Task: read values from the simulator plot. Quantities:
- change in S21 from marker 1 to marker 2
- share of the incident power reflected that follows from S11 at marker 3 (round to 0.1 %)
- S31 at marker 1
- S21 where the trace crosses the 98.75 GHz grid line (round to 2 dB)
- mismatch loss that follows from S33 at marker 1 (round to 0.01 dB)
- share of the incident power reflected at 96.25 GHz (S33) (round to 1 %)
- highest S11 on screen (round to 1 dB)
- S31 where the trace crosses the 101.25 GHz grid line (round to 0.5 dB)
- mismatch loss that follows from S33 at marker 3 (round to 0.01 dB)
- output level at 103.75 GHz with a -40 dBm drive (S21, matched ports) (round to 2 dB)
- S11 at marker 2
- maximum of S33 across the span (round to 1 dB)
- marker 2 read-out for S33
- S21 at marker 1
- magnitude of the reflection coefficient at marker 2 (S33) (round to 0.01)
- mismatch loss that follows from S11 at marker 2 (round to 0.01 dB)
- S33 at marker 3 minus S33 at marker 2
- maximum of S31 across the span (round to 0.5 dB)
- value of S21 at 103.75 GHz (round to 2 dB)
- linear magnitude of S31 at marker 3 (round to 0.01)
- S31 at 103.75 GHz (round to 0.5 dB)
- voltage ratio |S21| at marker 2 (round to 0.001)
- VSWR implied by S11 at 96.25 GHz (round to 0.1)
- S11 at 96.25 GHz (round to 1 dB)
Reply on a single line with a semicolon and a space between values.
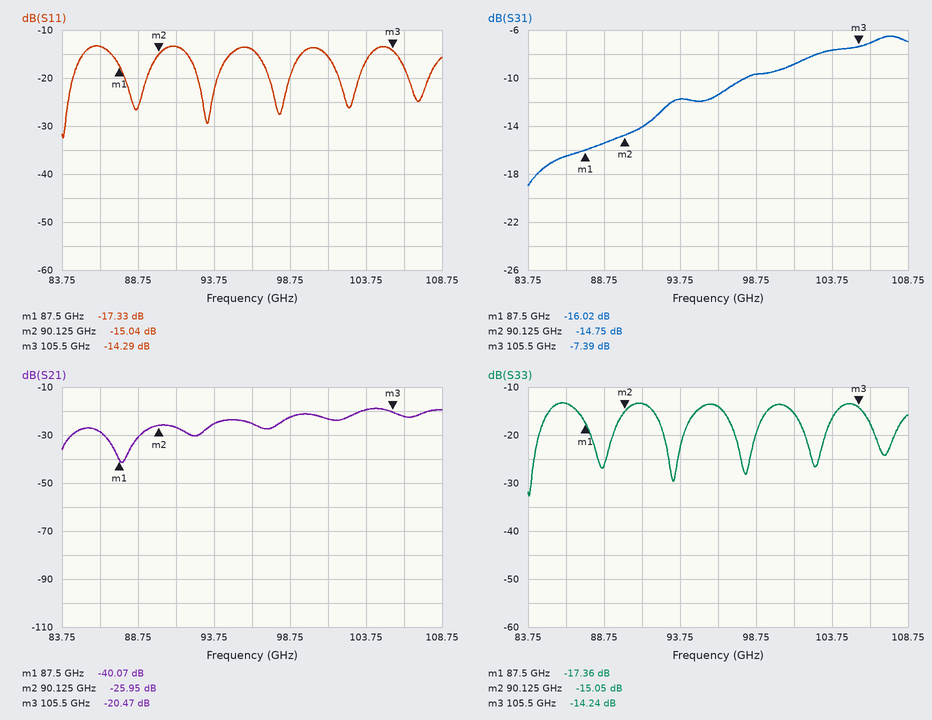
14.12 dB; 3.7 %; -16.02 dB; -22 dB; 0.08 dB; 4 %; -13 dB; -9.0 dB; 0.17 dB; -60 dBm; -15.04 dB; -13 dB; -15.05 dB; -40.07 dB; 0.18; 0.14 dB; 0.81 dB; -6.5 dB; -20 dB; 0.43; -7.5 dB; 0.050; 1.5; -14 dB
